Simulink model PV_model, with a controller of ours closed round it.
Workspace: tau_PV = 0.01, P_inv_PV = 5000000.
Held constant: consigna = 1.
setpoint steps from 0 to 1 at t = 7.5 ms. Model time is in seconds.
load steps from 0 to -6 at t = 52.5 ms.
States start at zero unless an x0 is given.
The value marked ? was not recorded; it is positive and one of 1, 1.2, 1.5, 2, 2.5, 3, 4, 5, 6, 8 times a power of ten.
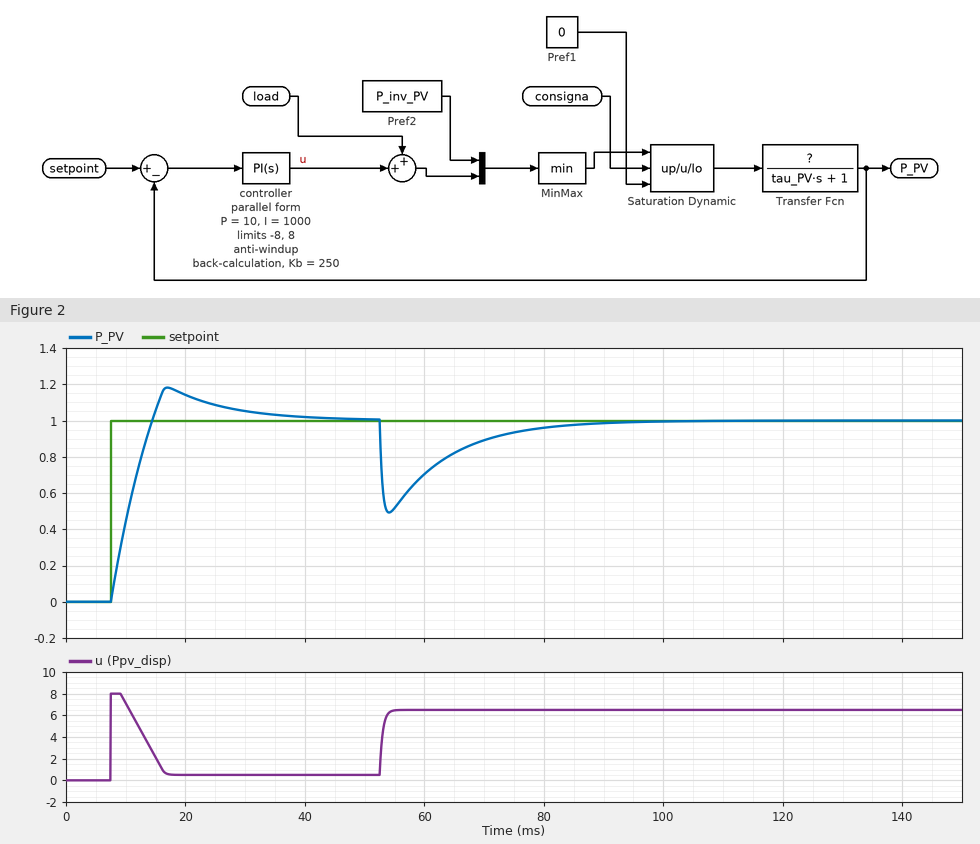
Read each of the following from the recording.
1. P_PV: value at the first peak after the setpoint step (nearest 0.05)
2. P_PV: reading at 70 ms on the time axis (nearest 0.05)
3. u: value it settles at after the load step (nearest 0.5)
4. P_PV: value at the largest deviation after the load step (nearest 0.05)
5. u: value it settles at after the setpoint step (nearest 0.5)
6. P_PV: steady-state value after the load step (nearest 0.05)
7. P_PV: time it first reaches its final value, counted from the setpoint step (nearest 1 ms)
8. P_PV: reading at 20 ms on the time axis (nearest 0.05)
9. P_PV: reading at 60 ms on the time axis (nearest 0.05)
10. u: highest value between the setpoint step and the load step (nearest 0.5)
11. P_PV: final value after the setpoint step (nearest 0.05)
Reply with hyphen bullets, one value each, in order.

- 1.20
- 0.90
- 6.5
- 0.50
- 0.5
- 1.00
- 7 ms
- 1.15
- 0.70
- 8.0
- 1.00
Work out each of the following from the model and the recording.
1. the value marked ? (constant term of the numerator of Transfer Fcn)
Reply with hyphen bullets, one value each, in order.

- 2
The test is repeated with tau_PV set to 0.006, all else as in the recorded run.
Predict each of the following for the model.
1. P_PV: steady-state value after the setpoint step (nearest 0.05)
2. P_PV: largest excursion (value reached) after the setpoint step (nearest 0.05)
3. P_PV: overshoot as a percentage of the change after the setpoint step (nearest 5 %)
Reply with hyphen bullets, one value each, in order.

- 1.00
- 1.10
- 10 %
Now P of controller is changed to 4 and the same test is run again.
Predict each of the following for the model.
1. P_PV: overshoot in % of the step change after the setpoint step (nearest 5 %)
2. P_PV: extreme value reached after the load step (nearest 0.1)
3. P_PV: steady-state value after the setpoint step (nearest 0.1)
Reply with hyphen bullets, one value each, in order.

- 35 %
- 0.0
- 1.0
